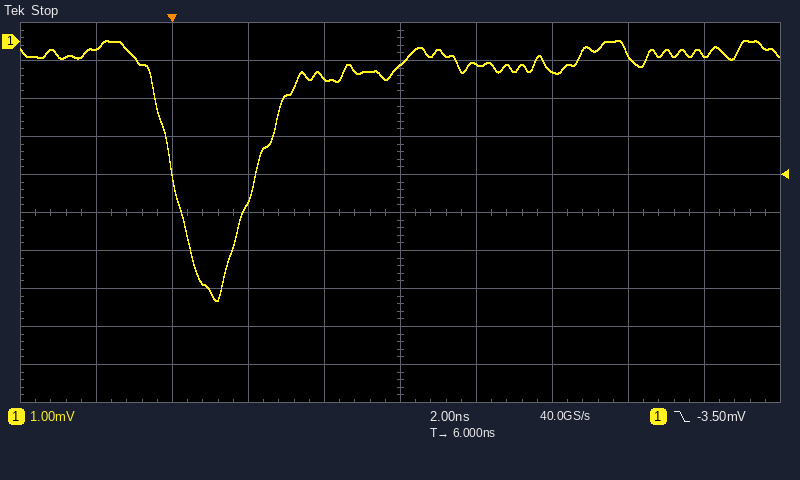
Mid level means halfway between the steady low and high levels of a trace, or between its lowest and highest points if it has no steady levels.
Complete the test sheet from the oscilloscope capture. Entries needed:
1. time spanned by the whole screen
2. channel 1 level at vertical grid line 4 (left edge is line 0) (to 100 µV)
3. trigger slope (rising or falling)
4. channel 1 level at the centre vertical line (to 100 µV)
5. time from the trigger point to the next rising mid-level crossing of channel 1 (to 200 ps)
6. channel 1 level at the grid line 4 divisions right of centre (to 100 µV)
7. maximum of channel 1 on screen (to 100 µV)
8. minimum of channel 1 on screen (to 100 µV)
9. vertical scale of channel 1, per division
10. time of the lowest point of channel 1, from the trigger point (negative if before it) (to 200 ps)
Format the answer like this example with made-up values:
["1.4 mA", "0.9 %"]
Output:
["20 ns", "-900 µV", "falling", "-600 µV", "2.2 ns", "-300 µV", "0.0 mV", "-6.8 mV", "1 mV", "+1.2 ns"]
